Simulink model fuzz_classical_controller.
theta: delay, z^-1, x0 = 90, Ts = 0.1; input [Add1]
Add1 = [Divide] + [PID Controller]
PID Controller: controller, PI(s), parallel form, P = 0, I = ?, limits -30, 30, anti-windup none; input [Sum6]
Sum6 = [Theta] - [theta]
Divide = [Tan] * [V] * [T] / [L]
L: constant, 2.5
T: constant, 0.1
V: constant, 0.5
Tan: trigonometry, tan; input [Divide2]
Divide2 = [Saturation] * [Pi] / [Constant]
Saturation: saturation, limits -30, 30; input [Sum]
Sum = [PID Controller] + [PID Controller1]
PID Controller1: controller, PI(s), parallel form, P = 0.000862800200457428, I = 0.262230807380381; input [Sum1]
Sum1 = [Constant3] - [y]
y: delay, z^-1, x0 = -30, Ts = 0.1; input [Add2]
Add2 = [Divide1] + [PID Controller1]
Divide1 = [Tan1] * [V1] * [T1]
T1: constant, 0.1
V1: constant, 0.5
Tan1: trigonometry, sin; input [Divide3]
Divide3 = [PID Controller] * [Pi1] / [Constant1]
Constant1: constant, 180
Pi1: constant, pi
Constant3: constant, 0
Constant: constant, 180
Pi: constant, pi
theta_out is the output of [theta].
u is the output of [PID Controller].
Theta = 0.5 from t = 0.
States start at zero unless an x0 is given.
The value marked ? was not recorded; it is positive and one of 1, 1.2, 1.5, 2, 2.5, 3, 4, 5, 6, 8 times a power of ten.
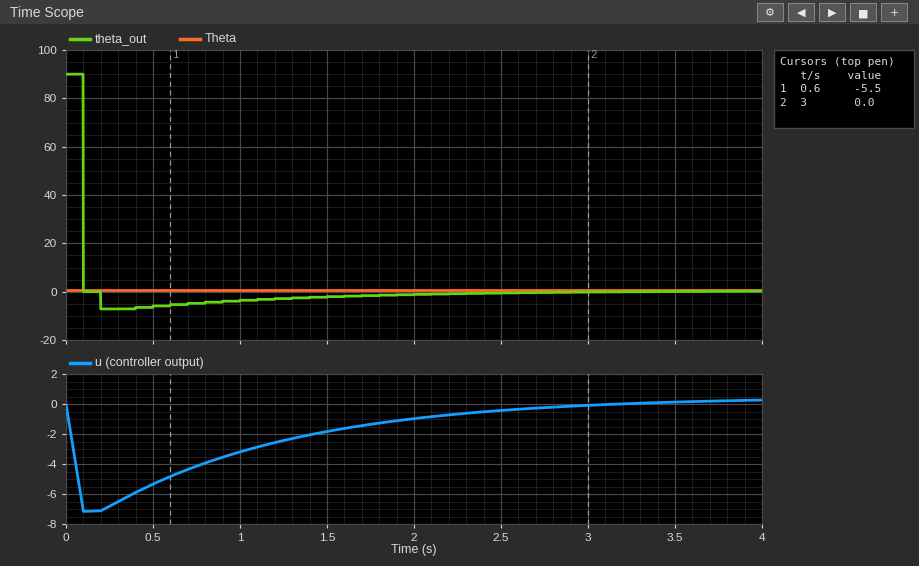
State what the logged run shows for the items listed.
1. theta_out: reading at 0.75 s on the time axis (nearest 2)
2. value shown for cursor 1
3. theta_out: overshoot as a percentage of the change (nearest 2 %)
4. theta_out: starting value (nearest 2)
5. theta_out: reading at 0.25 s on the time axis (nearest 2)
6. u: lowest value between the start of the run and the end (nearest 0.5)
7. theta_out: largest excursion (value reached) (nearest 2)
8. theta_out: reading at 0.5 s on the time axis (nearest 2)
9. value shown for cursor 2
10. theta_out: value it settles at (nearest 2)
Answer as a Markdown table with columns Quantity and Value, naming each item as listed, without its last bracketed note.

| Quantity | Value |
|---|---|
| theta_out: reading at 0.75 s on the time axis | -4 |
| value shown for cursor 1 | -5.5 |
| theta_out: overshoot as a percentage of the change | 8 % |
| theta_out: starting value | 90 |
| theta_out: reading at 0.25 s on the time axis | -8 |
| u: lowest value between the start of the run and the end | -7.0 |
| theta_out: largest excursion (value reached) | -8 |
| theta_out: reading at 0.5 s on the time axis | -6 |
| value shown for cursor 2 | 0.0 |
| theta_out: value it settles at | 0 |
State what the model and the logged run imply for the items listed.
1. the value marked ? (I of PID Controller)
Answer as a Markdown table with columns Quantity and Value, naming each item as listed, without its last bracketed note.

| Quantity | Value |
|---|---|
| the value marked ? | 0.8 |
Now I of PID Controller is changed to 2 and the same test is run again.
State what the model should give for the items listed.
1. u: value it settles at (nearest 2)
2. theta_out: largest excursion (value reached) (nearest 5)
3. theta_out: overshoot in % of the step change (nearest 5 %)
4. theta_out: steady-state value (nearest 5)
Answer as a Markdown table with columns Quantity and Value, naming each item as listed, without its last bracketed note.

| Quantity | Value |
|---|---|
| u: value it settles at | 0 |
| theta_out: largest excursion (value reached) | -20 |
| theta_out: overshoot in % of the step change | 20 % |
| theta_out: steady-state value | 0 |
